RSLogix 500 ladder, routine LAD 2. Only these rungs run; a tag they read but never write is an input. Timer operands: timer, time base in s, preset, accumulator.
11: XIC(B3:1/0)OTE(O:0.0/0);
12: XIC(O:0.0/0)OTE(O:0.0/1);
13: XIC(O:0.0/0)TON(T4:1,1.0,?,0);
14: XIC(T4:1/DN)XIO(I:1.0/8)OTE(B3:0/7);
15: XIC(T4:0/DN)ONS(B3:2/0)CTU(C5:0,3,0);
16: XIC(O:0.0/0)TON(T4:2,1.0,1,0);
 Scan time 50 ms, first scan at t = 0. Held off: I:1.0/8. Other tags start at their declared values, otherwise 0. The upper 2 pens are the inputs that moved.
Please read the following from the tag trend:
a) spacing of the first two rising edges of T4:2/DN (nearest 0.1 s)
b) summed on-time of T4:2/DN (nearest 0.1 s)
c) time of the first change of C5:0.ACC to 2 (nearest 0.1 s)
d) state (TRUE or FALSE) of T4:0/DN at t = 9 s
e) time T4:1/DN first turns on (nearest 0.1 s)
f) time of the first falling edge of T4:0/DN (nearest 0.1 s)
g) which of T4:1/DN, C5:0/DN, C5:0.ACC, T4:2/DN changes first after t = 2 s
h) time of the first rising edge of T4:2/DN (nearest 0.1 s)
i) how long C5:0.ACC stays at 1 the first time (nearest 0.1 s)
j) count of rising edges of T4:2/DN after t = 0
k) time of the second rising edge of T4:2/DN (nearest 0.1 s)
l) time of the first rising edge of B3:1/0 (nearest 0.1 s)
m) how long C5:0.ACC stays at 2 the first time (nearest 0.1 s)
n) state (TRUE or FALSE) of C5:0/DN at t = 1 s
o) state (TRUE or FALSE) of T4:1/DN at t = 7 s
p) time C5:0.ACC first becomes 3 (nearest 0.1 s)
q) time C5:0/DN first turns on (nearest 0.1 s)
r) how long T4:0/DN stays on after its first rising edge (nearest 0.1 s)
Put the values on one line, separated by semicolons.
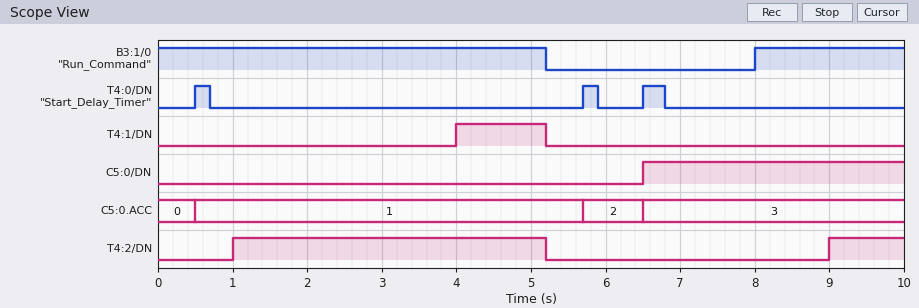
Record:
8.0 s; 5.2 s; 5.7 s; FALSE; 4.0 s; 0.7 s; T4:1/DN; 1.0 s; 5.2 s; 2; 9.0 s; 8.0 s; 0.8 s; FALSE; FALSE; 6.5 s; 6.5 s; 0.2 s
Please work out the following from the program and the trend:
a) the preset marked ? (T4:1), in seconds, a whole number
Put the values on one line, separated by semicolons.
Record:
4 s
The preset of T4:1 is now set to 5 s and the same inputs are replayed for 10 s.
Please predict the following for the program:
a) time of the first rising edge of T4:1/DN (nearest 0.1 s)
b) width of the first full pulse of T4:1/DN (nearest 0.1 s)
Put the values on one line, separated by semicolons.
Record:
5.0 s; 0.2 s
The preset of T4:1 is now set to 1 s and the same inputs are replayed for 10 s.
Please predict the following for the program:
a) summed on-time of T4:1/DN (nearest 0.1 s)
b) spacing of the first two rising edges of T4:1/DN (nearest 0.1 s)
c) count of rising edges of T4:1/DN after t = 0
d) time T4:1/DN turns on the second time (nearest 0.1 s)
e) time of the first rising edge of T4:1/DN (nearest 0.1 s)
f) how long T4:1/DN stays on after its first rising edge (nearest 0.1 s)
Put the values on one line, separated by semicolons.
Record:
5.2 s; 8.0 s; 2; 9.0 s; 1.0 s; 4.2 s
